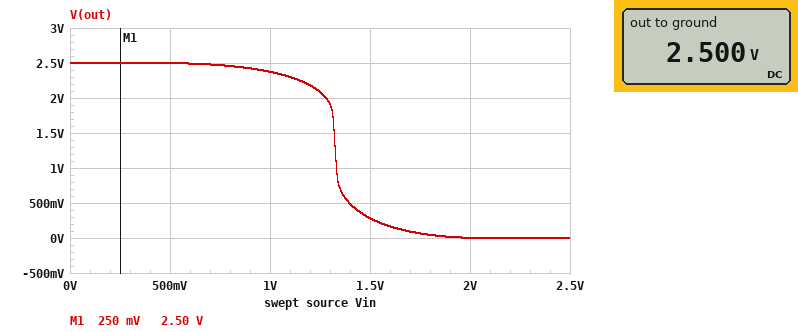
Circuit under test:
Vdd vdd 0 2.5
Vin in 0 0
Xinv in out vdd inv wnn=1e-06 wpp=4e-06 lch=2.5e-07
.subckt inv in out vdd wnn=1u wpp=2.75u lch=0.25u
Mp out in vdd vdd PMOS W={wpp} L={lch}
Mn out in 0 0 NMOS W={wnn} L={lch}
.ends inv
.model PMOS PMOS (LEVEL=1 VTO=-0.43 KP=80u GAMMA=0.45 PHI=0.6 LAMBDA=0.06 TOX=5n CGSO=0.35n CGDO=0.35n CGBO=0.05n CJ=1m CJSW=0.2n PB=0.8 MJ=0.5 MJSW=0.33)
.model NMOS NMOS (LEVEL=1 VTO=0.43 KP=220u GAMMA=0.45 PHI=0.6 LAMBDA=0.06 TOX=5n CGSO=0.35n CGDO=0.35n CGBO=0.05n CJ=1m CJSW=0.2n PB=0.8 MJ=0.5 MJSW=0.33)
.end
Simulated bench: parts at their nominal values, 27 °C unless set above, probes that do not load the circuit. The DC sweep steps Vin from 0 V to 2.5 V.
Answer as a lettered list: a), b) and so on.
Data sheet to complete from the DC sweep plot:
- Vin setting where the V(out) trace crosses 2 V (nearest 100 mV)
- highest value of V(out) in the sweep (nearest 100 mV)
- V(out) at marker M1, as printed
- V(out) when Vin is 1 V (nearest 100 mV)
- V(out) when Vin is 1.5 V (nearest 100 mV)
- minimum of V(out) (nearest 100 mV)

a) 1.3 V
b) 2.5 V
c) 2.50 V
d) 2.4 V
e) 300 mV
f) 0 V
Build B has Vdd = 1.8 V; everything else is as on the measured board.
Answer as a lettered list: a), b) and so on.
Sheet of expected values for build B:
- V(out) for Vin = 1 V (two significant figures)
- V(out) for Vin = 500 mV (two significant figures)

a) 240 mV
b) 1.8 V
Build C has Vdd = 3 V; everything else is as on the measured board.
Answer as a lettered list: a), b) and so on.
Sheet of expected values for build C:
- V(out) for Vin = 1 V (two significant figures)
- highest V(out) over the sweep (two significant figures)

a) 2.9 V
b) 3.0 V
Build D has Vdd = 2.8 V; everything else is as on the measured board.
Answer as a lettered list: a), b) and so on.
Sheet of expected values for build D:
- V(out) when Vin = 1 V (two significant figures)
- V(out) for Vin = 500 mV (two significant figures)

a) 2.7 V
b) 2.8 V
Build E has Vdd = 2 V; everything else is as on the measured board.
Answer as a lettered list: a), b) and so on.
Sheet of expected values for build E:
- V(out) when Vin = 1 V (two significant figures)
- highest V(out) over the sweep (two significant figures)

a) 1.7 V
b) 2.0 V
